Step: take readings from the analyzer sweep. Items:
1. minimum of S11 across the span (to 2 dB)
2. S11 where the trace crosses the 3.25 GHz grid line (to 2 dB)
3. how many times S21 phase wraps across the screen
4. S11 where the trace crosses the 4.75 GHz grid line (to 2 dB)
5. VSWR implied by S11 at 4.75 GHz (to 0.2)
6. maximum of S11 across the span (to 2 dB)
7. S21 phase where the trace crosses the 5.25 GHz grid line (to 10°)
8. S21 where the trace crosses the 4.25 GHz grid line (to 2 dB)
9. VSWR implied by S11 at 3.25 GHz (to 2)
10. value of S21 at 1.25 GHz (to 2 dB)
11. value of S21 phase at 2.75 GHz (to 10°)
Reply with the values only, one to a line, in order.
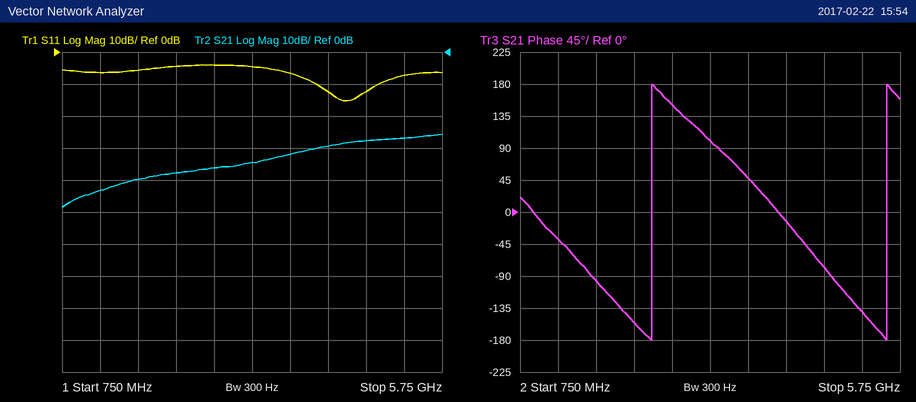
-16 dB
-4 dB
2
-12 dB
1.6
-4 dB
-140°
-30 dB
4
-44 dB
150°
